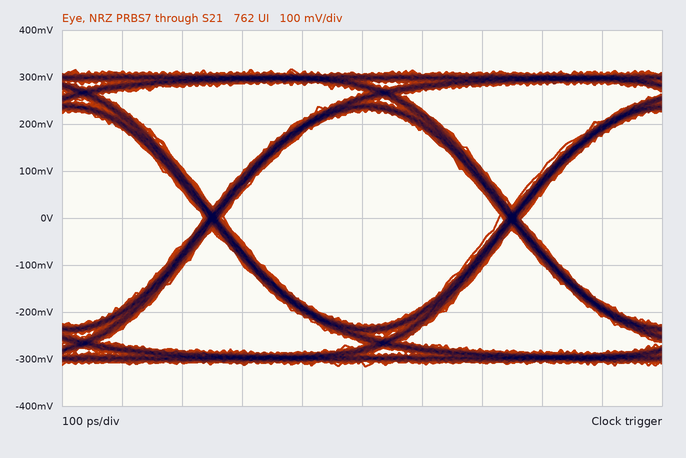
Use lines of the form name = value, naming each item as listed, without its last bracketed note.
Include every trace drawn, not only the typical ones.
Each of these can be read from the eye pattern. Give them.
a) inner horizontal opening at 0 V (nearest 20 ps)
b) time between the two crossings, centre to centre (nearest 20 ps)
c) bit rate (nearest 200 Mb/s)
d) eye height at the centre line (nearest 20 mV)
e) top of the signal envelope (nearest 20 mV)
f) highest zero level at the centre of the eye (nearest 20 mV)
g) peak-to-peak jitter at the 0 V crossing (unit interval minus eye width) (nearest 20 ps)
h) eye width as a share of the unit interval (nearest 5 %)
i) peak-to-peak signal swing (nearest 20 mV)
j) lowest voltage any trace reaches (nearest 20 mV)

inner horizontal opening at 0 V = 460 ps
time between the two crossings, centre to centre = 500 ps
bit rate = 2.0 Gb/s
eye height at the centre line = 460 mV
top of the signal envelope = 320 mV
highest zero level at the centre of the eye = -220 mV
peak-to-peak jitter at the 0 V crossing (unit interval minus eye width) = 40 ps
eye width as a share of the unit interval = 90 %
peak-to-peak signal swing = 640 mV
lowest voltage any trace reaches = -320 mV
